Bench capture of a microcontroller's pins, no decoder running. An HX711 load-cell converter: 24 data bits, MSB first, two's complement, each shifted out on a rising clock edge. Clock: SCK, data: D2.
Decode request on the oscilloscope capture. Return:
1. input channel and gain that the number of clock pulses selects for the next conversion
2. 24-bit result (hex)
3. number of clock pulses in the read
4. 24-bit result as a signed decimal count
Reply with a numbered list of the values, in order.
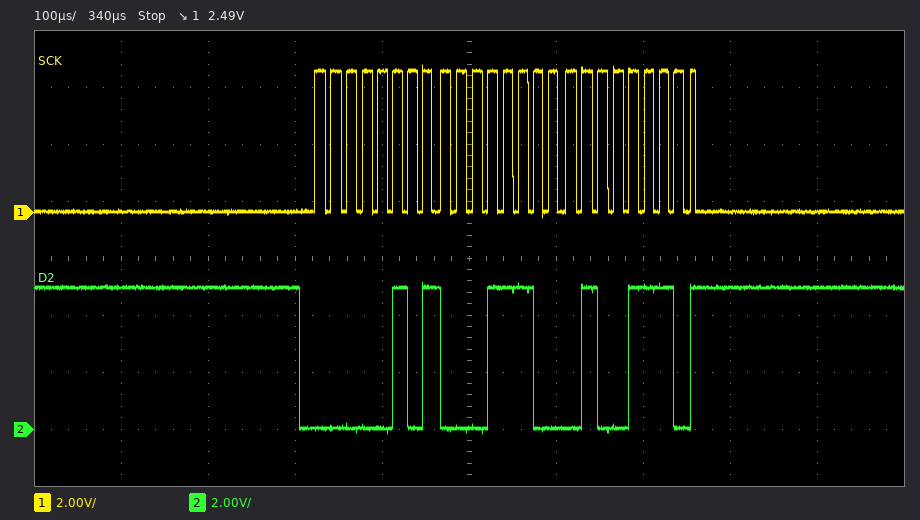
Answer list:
1. channel A, gain 128
2. 0x051C4E
3. 25
4. 334926
